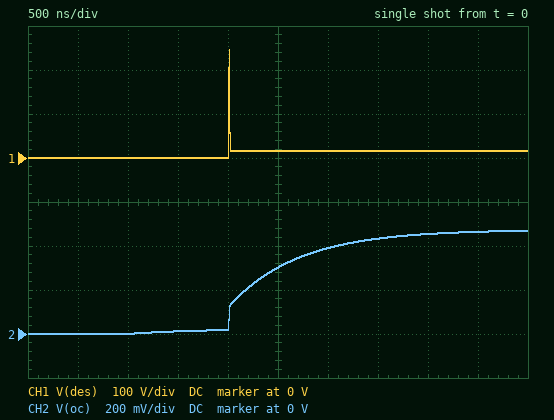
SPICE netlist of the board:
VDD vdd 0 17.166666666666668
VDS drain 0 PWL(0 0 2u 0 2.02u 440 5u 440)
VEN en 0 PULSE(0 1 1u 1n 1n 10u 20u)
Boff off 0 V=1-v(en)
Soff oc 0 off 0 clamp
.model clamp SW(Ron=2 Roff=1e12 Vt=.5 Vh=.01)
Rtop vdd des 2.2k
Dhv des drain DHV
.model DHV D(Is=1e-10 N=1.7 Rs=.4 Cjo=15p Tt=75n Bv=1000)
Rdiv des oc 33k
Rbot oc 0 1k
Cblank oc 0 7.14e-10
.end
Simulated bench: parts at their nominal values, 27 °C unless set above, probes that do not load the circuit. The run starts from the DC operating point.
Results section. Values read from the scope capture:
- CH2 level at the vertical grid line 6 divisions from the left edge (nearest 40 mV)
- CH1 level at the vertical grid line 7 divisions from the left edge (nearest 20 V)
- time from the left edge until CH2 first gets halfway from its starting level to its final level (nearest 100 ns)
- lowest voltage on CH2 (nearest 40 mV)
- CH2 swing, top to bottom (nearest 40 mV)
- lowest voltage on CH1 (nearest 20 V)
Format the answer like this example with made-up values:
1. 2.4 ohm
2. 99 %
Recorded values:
1. 400 mV
2. 20 V
3. 2.3 µs
4. 0 V
5. 480 mV
6. 0 V
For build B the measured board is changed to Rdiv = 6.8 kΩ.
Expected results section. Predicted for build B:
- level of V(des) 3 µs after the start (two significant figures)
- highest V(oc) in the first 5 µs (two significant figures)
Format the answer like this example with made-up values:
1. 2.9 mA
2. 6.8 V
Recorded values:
1. 13 V
2. 1.7 V
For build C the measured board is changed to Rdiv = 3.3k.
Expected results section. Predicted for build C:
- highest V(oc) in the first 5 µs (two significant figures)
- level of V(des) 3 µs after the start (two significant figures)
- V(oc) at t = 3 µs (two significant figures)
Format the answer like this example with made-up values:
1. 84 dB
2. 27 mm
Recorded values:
1. 2.6 V
2. 11 V
3. 2.3 V
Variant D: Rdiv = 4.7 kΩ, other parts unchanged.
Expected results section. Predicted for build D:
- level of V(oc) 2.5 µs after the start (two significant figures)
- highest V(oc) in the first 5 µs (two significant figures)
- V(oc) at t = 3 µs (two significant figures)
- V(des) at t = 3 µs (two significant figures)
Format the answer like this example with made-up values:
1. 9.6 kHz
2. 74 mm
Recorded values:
1. 1.5 V
2. 2.2 V
3. 1.9 V
4. 12 V
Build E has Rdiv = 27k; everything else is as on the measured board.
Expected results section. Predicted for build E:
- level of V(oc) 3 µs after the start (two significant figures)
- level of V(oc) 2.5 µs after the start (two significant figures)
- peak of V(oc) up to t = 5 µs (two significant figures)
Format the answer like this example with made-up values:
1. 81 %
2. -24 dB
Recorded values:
1. 470 mV
2. 360 mV
3. 560 mV
